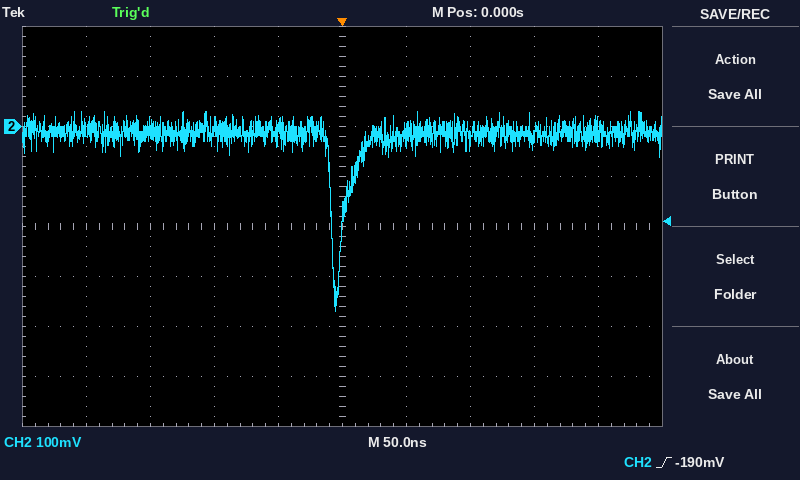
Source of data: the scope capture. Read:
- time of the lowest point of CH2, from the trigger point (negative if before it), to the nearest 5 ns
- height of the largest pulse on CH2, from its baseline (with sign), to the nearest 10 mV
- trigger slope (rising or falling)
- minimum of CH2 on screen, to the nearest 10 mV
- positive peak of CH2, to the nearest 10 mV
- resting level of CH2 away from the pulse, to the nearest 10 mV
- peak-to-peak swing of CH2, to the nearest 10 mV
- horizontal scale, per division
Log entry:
-5 ns
-360 mV
rising
-370 mV
30 mV
-10 mV
400 mV
50 ns
